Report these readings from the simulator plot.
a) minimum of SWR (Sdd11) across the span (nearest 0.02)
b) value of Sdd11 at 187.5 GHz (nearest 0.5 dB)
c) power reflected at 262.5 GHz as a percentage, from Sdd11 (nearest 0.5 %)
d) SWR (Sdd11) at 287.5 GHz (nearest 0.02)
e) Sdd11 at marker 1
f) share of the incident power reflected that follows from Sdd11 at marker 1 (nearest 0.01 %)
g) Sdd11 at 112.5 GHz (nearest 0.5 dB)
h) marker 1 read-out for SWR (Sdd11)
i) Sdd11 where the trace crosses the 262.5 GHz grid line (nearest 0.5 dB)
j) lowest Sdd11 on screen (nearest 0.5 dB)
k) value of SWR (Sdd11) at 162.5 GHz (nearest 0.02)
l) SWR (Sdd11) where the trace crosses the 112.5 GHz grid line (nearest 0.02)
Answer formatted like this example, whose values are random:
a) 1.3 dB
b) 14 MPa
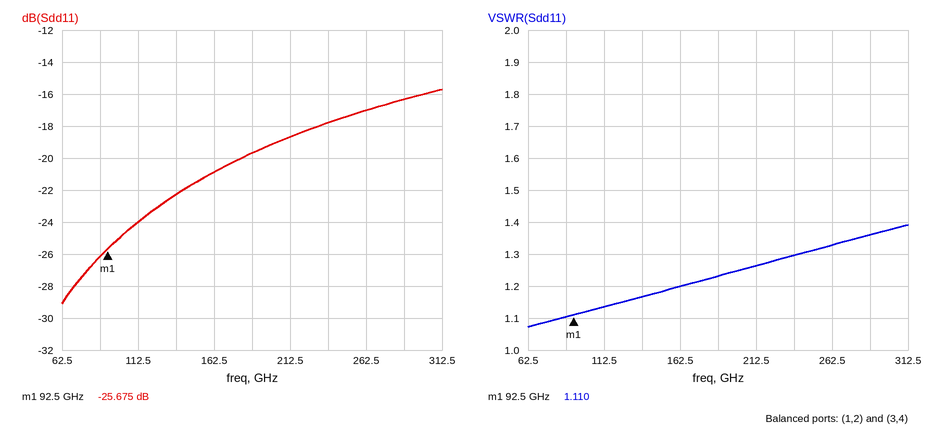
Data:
a) 1.08
b) -19.5 dB
c) 2.0 %
d) 1.36
e) -25.675 dB
f) 0.27 %
g) -24.0 dB
h) 1.110
i) -17.0 dB
j) -29.0 dB
k) 1.20
l) 1.14
